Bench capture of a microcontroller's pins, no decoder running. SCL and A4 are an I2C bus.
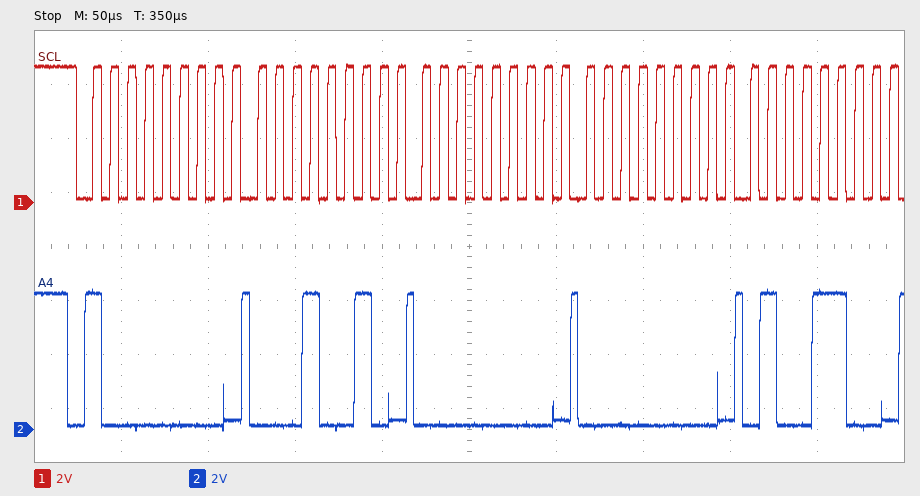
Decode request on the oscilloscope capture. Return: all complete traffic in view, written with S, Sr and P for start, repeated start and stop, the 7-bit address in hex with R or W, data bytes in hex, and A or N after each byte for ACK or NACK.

S 40W A 12 A 00 A 00 A 4C A
